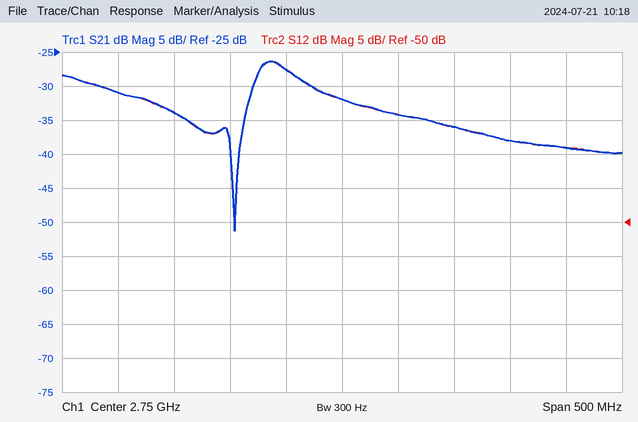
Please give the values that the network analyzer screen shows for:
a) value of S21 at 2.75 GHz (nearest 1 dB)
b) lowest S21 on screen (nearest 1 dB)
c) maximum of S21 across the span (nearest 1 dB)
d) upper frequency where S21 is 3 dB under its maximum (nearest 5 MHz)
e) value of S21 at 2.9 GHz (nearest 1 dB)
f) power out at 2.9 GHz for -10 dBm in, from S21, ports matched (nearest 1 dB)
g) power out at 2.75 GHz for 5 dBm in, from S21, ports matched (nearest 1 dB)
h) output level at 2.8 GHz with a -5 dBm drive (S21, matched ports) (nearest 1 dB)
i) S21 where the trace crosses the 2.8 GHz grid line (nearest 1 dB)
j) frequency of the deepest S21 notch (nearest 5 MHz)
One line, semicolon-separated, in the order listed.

-32 dB; -51 dB; -26 dB; 2.715 GHz; -38 dB; -48 dBm; -27 dBm; -39 dBm; -34 dB; 2.655 GHz
